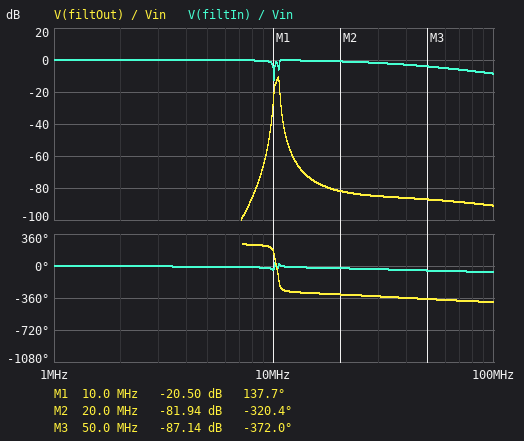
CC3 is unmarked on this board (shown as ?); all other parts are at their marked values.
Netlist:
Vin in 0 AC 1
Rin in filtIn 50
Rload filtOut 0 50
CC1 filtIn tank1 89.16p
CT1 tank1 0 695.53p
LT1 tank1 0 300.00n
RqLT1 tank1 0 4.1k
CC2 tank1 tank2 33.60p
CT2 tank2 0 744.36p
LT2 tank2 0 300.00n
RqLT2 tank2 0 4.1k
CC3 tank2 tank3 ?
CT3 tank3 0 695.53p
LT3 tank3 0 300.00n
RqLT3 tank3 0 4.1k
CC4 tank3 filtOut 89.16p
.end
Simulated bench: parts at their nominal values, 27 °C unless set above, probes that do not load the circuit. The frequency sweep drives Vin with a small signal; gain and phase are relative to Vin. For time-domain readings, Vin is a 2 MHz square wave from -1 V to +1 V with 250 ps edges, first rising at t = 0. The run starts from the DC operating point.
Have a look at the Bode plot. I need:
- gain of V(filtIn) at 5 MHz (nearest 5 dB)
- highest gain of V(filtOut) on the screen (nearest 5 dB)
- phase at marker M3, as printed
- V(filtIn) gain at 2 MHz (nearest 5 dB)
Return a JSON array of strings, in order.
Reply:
["0 dB", "-10 dB", "-372.0 deg", "0 dB"]
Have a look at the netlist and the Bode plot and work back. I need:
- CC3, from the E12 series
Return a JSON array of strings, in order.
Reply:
["12 pF"]
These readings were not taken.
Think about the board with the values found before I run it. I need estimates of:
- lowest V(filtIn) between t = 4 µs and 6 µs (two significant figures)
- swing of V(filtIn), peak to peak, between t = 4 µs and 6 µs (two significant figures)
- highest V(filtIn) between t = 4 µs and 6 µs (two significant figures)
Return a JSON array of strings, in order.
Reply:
["-1.2 V", "2.4 V", "1.2 V"]
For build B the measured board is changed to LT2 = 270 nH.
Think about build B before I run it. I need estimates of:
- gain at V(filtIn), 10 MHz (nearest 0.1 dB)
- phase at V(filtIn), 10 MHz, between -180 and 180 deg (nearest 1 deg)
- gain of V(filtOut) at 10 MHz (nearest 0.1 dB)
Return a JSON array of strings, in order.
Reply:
["-6.2 dB", "-51 deg", "-30.9 dB"]
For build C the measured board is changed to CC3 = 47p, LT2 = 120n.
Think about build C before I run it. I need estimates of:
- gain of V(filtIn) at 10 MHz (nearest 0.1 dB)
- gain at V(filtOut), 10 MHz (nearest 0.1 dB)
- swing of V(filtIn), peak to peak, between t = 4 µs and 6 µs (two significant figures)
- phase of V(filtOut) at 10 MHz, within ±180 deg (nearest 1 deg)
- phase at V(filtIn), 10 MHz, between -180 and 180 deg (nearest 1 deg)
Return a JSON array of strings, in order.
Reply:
["-4.6 dB", "-33.5 dB", "2.3 V", "141 deg", "-47 deg"]
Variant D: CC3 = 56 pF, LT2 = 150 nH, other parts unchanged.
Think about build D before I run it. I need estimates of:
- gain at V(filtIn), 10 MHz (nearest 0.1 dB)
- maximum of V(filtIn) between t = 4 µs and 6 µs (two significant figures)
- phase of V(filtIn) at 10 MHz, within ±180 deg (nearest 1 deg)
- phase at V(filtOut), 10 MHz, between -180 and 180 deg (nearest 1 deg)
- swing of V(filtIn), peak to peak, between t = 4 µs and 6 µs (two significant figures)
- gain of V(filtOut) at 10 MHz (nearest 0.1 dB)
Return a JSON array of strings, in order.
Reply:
["-4.7 dB", "1.2 V", "-47 deg", "121 deg", "2.3 V", "-27.1 dB"]
